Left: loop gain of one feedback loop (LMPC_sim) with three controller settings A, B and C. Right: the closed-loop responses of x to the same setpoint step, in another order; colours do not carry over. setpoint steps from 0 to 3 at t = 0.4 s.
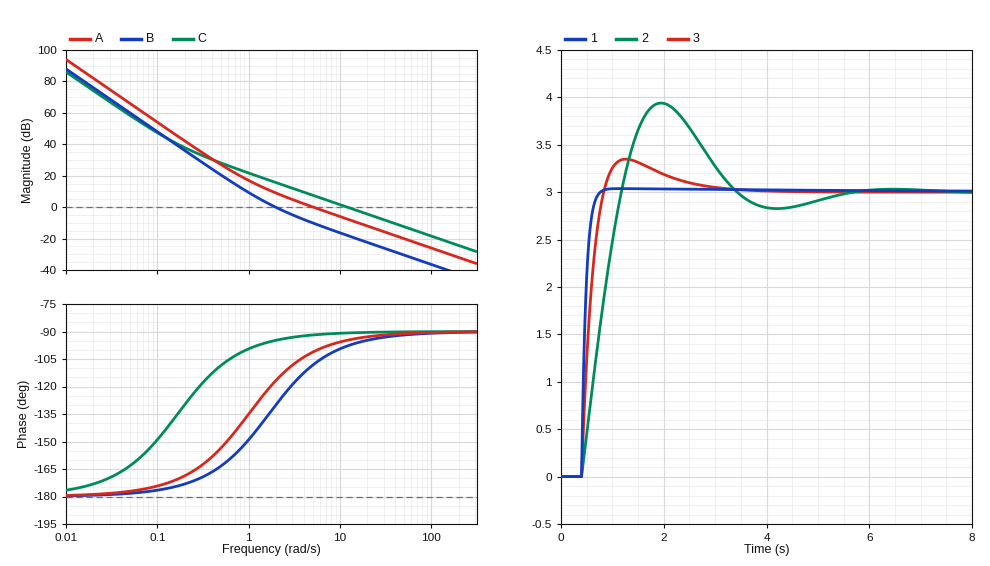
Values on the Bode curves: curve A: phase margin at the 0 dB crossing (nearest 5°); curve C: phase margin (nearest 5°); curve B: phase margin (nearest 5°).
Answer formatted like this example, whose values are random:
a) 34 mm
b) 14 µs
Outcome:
a) 80°
b) 90°
c) 50°
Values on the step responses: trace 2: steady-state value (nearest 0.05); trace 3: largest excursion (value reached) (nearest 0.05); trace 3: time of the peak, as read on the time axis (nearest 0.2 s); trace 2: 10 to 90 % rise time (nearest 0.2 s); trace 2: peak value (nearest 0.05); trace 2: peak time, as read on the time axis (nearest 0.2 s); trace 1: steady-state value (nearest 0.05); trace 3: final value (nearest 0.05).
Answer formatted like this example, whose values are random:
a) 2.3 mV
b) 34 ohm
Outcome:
a) 3.00
b) 3.35
c) 1.2 s
d) 0.6 s
e) 3.95
f) 2.0 s
g) 3.00
h) 3.00
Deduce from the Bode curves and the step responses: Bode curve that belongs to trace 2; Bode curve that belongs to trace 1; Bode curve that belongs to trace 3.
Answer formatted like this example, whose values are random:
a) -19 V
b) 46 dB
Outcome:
a) B
b) C
c) A
